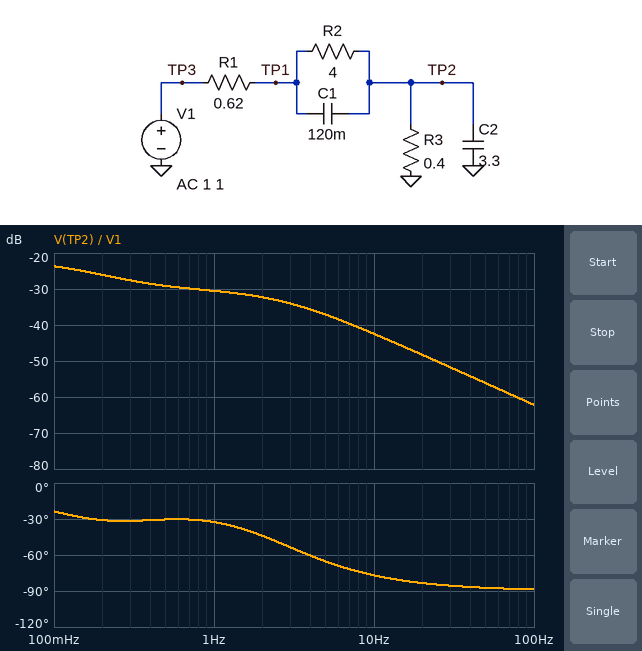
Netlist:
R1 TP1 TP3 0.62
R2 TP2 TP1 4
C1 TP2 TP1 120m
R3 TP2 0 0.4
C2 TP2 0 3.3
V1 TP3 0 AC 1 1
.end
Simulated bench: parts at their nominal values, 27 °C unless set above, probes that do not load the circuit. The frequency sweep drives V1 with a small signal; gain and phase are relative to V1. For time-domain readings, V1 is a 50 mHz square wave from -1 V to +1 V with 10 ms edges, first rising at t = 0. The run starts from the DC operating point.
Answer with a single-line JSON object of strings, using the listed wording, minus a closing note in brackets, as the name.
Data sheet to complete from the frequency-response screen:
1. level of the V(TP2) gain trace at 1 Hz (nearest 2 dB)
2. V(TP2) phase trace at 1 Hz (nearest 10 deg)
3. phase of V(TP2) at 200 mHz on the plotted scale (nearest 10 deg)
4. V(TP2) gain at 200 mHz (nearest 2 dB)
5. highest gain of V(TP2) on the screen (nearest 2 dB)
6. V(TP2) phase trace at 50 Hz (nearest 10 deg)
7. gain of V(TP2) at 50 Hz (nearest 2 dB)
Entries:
{"level of the V(TP2) gain trace at 1 Hz": "-30 dB", "V(TP2) phase trace at 1 Hz": "-30 deg", "phase of V(TP2) at 200 mHz on the plotted scale": "-30 deg", "V(TP2) gain at 200 mHz": "-26 dB", "highest gain of V(TP2) on the screen": "-24 dB", "V(TP2) phase trace at 50 Hz": "-90 deg", "gain of V(TP2) at 50 Hz": "-56 dB"}
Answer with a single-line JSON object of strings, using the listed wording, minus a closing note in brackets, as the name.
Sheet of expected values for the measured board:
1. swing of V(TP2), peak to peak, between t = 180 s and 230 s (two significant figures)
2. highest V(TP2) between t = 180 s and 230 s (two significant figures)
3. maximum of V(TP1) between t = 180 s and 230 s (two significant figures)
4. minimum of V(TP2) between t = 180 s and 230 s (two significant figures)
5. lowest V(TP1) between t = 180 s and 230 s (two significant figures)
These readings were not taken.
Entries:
{"swing of V(TP2), peak to peak, between t = 180 s and 230 s": "160 mV", "highest V(TP2) between t = 180 s and 230 s": "80 mV", "maximum of V(TP1) between t = 180 s and 230 s": "880 mV", "minimum of V(TP2) between t = 180 s and 230 s": "-80 mV", "lowest V(TP1) between t = 180 s and 230 s": "-880 mV"}
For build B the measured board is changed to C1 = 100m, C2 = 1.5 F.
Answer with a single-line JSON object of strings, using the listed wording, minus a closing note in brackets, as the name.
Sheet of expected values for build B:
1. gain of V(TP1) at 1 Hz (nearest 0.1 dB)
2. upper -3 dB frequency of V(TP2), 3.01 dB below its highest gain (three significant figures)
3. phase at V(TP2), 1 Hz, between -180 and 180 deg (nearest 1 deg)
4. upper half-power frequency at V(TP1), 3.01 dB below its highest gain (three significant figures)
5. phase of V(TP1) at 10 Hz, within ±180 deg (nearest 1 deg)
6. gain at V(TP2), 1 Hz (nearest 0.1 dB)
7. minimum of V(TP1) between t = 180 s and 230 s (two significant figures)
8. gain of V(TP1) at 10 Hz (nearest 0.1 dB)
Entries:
{"gain of V(TP1) at 1 Hz": "-1.6 dB", "upper -3 dB frequency of V(TP2), 3.01 dB below its highest gain": "771 mHz", "phase at V(TP2), 1 Hz, between -180 and 180 deg": "-24 deg", "upper half-power frequency at V(TP1), 3.01 dB below its highest gain": "3.12 Hz", "phase of V(TP1) at 10 Hz, within ±180 deg": "-73 deg", "gain at V(TP2), 1 Hz": "-25.3 dB", "minimum of V(TP1) between t = 180 s and 230 s": "-880 mV", "gain of V(TP1) at 10 Hz": "-11.7 dB"}
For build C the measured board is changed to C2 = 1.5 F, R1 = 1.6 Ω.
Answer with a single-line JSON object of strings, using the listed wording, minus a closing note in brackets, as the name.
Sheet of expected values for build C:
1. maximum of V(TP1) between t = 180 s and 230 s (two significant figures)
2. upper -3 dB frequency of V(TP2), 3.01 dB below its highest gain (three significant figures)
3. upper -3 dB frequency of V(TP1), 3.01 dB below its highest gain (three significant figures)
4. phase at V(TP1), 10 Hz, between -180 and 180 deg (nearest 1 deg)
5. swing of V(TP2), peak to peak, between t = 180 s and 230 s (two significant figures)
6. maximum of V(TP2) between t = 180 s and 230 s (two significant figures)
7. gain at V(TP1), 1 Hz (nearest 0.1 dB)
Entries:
{"maximum of V(TP1) between t = 180 s and 230 s": "730 mV", "upper -3 dB frequency of V(TP2), 3.01 dB below its highest gain": "771 mHz", "upper -3 dB frequency of V(TP1), 3.01 dB below its highest gain": "1.22 Hz", "phase at V(TP1), 10 Hz, between -180 and 180 deg": "-83 deg", "swing of V(TP2), peak to peak, between t = 180 s and 230 s": "130 mV", "maximum of V(TP2) between t = 180 s and 230 s": "67 mV", "gain at V(TP1), 1 Hz": "-4.9 dB"}
